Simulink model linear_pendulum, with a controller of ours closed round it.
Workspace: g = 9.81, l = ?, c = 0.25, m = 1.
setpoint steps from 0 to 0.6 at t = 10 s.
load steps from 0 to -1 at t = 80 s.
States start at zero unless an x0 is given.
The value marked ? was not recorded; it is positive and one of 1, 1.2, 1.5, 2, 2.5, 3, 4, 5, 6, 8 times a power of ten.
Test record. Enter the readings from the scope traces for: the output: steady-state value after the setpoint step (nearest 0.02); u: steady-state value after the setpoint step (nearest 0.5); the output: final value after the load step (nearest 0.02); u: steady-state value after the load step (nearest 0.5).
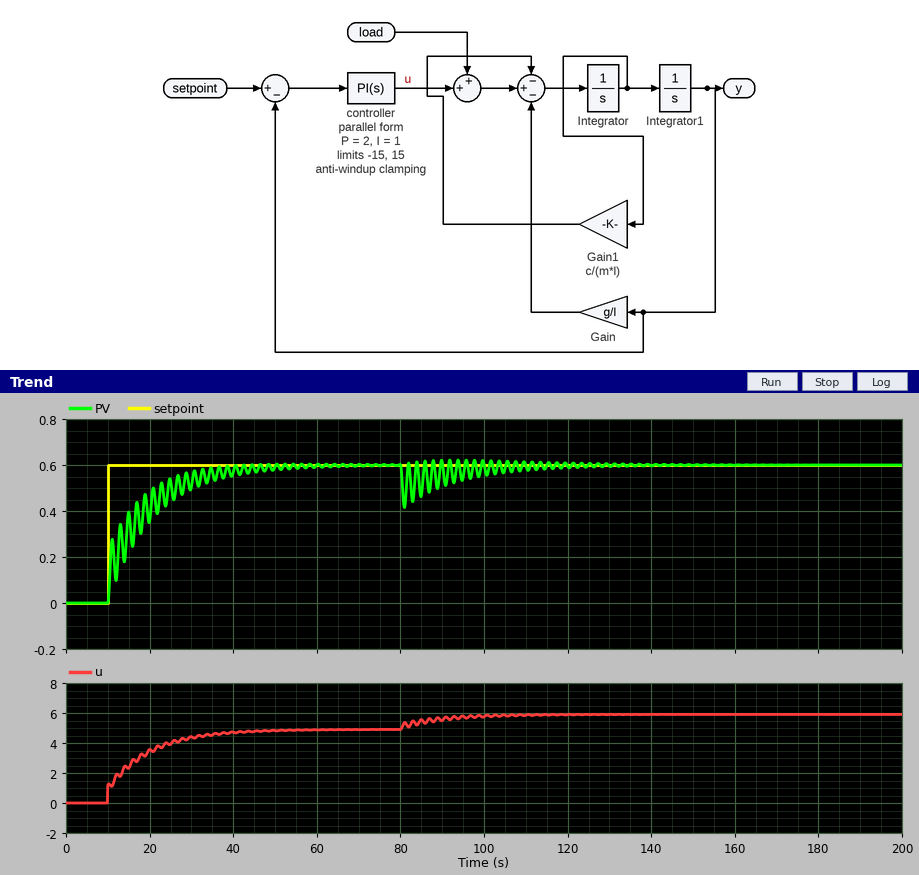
0.60
5.0
0.60
6.0
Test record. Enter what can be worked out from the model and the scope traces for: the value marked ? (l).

1.2
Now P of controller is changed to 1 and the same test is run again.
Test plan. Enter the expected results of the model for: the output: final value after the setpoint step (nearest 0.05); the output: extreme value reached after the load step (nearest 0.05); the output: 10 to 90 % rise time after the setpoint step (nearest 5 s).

0.60
0.40
15 s
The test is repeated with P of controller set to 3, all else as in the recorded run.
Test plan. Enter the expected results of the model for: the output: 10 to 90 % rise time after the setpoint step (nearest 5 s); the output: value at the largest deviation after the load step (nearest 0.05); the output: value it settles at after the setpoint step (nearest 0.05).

15 s
0.45
0.60
